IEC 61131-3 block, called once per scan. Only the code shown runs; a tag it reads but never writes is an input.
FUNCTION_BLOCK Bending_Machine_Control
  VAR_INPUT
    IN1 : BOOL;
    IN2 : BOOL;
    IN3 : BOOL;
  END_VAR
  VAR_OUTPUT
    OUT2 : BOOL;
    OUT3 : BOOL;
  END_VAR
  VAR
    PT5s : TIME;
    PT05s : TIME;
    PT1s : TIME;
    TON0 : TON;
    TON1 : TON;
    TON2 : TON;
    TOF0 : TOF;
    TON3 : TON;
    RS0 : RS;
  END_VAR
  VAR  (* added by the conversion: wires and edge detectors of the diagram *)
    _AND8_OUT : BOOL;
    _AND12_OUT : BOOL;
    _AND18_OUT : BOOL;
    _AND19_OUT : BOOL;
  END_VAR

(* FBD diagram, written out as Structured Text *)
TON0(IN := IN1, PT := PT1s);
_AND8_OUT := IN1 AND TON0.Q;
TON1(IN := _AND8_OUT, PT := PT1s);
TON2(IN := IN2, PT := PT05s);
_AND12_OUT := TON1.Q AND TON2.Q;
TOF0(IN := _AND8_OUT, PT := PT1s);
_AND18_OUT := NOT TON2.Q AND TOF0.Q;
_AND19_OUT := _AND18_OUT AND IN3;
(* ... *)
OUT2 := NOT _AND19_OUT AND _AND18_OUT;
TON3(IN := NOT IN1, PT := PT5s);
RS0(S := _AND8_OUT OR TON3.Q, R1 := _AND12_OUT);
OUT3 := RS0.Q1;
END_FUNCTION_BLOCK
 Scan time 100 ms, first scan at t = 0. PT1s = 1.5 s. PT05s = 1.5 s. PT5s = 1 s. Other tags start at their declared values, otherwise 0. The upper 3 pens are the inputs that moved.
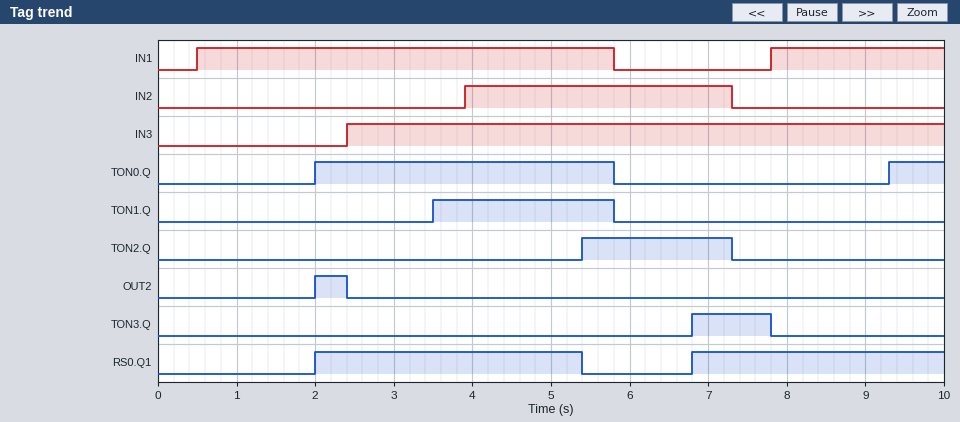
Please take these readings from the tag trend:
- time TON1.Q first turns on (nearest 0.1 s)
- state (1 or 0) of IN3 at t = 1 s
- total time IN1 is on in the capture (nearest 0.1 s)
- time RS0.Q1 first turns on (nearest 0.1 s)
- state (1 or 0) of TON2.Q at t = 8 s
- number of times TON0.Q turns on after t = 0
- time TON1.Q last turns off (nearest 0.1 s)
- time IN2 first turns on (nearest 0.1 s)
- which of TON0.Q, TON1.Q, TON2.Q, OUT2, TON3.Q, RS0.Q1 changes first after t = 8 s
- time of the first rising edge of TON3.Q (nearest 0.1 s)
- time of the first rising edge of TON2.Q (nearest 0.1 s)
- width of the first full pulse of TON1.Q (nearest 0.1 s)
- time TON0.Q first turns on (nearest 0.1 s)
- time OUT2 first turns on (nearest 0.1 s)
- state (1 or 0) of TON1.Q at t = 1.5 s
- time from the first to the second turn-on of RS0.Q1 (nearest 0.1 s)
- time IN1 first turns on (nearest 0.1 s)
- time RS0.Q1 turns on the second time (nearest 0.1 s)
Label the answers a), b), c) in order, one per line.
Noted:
a) 3.5 s
b) 0
c) 7.5 s
d) 2.0 s
e) 0
f) 2
g) 5.8 s
h) 3.9 s
i) TON0.Q
j) 6.8 s
k) 5.4 s
l) 2.3 s
m) 2.0 s
n) 2.0 s
o) 0
p) 4.8 s
q) 0.5 s
r) 6.8 s
